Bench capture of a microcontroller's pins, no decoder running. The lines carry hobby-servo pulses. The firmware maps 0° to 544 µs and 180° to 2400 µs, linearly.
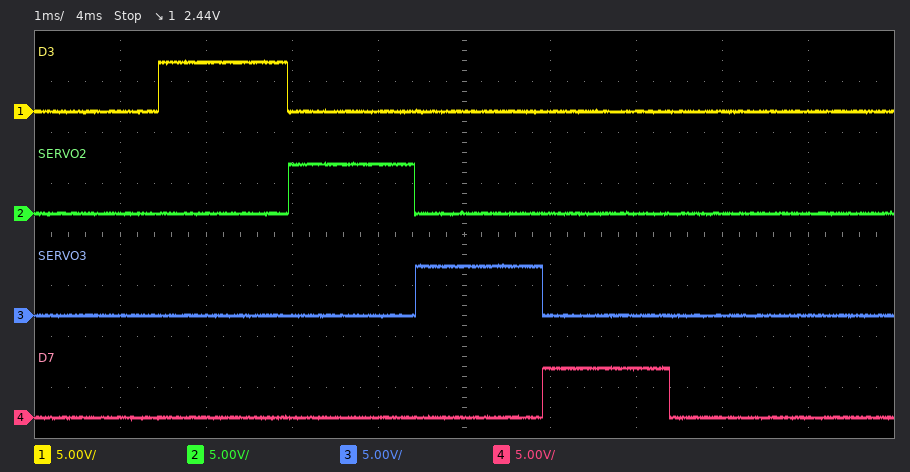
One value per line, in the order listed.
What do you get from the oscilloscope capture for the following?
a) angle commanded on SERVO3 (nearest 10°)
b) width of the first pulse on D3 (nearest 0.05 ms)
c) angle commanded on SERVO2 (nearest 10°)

90°
1.50 ms
90°
